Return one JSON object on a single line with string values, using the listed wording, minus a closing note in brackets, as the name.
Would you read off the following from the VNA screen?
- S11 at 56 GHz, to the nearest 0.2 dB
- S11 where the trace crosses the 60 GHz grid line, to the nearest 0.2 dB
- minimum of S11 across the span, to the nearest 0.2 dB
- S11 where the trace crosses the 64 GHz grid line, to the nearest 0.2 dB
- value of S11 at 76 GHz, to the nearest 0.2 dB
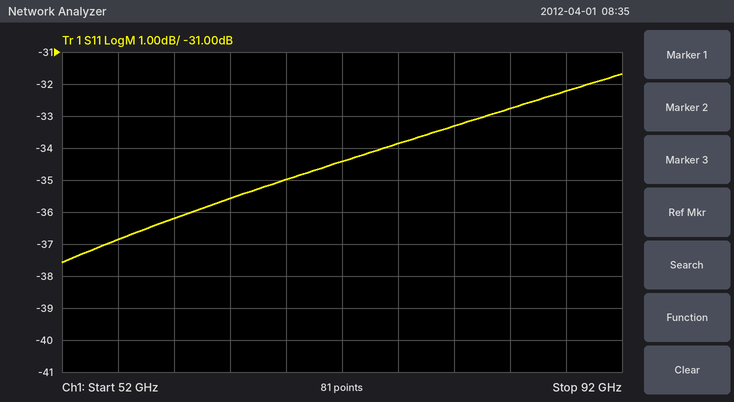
{"S11 at 56 GHz, to the nearest 0.2 dB": "-36.8 dB", "S11 where the trace crosses the 60 GHz grid line, to the nearest 0.2 dB": "-36.2 dB", "minimum of S11 across the span, to the nearest 0.2 dB": "-37.6 dB", "S11 where the trace crosses the 64 GHz grid line, to the nearest 0.2 dB": "-35.6 dB", "value of S11 at 76 GHz, to the nearest 0.2 dB": "-33.8 dB"}
